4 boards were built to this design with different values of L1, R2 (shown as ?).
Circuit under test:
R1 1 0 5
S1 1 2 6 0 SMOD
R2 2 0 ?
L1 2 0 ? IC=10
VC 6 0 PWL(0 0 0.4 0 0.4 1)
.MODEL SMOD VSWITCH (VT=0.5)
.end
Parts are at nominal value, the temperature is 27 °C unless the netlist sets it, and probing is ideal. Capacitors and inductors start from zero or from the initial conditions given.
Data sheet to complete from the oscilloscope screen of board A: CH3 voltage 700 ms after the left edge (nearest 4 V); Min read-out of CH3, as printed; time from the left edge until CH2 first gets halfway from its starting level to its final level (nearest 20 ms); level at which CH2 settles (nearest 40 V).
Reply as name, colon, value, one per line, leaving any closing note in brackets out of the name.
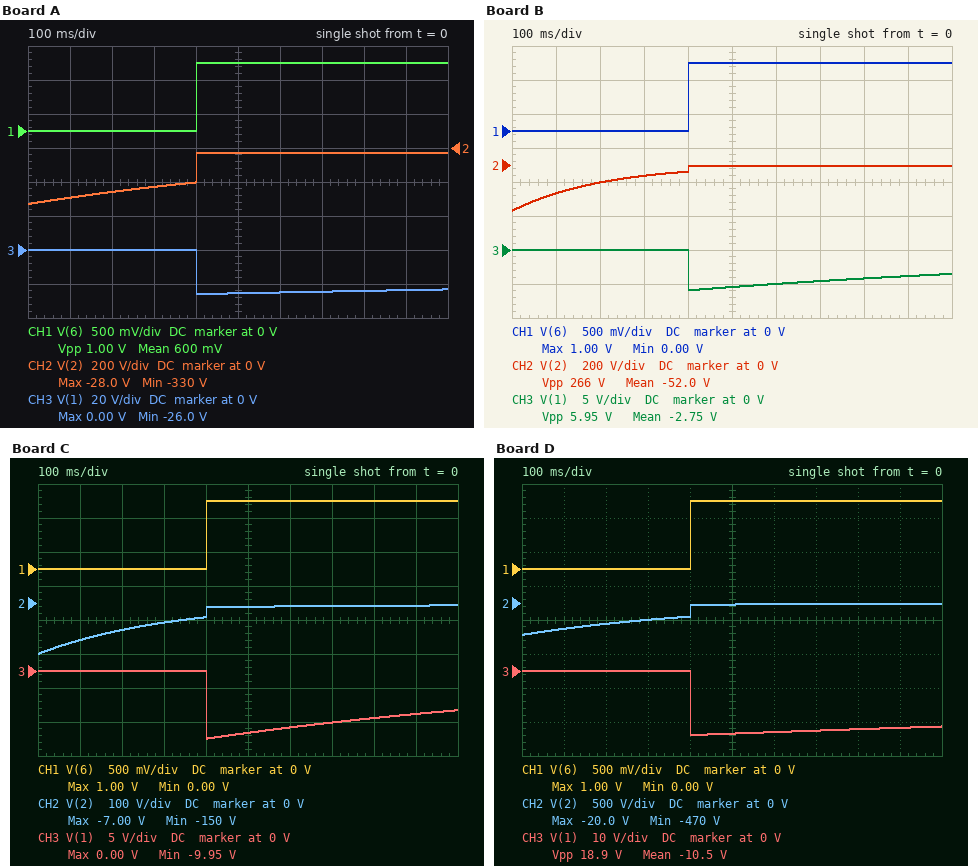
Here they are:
CH3 voltage 700 ms after the left edge: -24 V
Min read-out of CH3, as printed: -26.0 V
time from the left edge until CH2 first gets halfway from its starting level to its final level: 400 ms
level at which CH2 settles: -40 V
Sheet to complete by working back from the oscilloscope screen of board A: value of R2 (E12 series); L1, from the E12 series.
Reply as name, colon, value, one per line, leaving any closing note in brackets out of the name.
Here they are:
value of R2: 33 Ω
L1, from the E12 series: 27 H
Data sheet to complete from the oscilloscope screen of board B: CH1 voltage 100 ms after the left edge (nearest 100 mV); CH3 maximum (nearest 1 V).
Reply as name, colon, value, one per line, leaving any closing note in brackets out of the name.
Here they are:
CH1 voltage 100 ms after the left edge: 0 V
CH3 maximum: 0 V
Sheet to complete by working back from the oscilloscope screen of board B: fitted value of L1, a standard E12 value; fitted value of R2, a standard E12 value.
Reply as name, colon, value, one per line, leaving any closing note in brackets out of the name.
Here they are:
fitted value of L1, a standard E12 value: 5.6 H
fitted value of R2, a standard E12 value: 27 Ω
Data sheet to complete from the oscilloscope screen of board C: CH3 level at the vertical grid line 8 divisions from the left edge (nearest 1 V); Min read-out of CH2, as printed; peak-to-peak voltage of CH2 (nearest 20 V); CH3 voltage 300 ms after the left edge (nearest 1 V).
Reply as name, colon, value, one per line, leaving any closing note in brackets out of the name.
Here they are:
CH3 level at the vertical grid line 8 divisions from the left edge: -7 V
Min read-out of CH2, as printed: -150 V
peak-to-peak voltage of CH2: 140 V
CH3 voltage 300 ms after the left edge: 0 V
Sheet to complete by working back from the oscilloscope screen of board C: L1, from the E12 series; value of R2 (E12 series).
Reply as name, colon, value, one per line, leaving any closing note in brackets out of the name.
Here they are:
L1, from the E12 series: 4.7 H
value of R2: 15 Ω
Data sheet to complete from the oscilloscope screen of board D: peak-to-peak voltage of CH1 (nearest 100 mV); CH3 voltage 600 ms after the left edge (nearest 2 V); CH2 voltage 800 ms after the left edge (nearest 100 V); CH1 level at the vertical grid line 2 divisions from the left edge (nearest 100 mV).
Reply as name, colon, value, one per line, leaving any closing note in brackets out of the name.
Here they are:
peak-to-peak voltage of CH1: 1.0 V
CH3 voltage 600 ms after the left edge: -18 V
CH2 voltage 800 ms after the left edge: 0 V
CH1 level at the vertical grid line 2 divisions from the left edge: 0 V
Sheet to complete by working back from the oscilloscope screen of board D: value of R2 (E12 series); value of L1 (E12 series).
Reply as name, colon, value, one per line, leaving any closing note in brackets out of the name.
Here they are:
value of R2: 47 Ω
value of L1: 22 H
